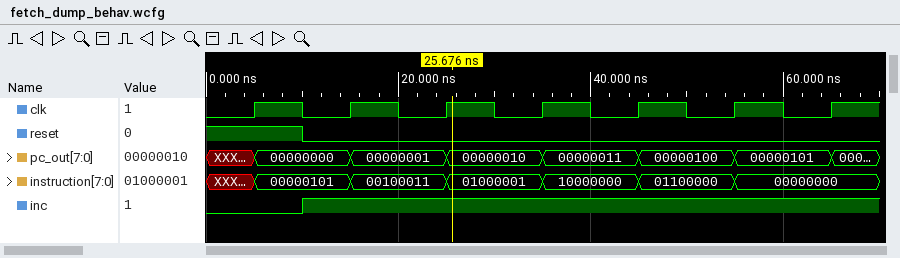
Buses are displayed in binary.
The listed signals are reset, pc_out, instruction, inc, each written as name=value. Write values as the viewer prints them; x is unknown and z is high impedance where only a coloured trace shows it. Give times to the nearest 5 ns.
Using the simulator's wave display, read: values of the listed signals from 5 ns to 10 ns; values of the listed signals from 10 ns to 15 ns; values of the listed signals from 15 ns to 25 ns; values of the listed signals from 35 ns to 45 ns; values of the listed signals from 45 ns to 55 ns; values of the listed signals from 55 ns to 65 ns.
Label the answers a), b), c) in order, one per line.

a) reset=1, pc_out=00000000, instruction=00000101, inc=0
b) reset=0, pc_out=00000000, instruction=00000101, inc=1
c) reset=0, pc_out=00000001, instruction=00100011, inc=1
d) reset=0, pc_out=00000011, instruction=10000000, inc=1
e) reset=0, pc_out=00000100, instruction=01100000, inc=1
f) reset=0, pc_out=00000101, instruction=00000000, inc=1
